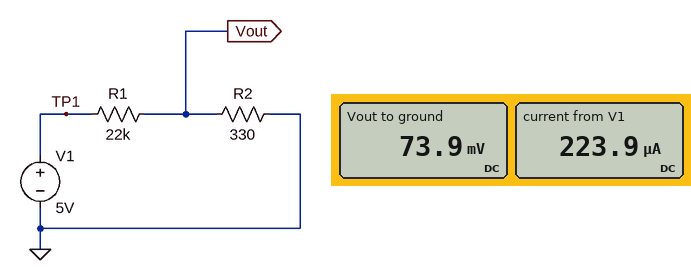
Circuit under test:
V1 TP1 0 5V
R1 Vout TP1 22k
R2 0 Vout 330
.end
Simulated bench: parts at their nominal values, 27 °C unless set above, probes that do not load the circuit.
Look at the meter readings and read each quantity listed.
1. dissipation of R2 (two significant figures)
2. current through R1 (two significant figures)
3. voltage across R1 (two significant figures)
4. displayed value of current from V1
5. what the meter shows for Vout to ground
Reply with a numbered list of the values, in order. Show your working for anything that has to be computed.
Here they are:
1. (73.9 mV)^2 / 330 Ω = 17 µW
2. (5 V - 73.9 mV) / 22 kΩ = 220 µA
3. 5 V - 73.9 mV = 4.9 V
4. 223.9 µA
5. 73.9 mV
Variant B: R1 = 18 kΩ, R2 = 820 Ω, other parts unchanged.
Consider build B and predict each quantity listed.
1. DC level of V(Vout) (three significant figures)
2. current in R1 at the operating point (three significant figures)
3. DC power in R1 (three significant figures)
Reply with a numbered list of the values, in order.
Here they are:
1. 218 mV
2. 266 µA
3. 1.27 mW
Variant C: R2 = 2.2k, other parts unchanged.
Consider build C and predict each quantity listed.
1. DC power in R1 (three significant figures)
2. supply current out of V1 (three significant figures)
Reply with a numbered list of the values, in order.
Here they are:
1. 939 µW
2. 207 µA
